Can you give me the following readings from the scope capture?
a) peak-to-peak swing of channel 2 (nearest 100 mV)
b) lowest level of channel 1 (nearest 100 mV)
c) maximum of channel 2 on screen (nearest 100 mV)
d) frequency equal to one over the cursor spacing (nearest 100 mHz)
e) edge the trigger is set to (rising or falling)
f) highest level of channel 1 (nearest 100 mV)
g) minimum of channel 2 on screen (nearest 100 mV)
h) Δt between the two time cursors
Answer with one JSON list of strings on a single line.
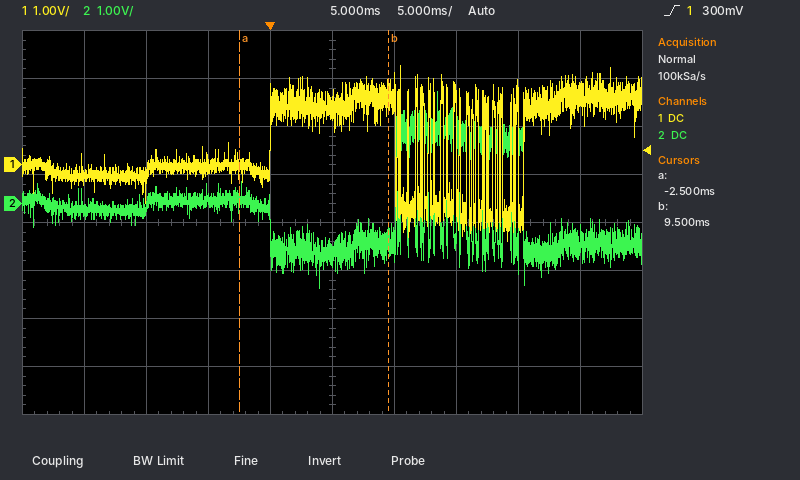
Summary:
["4.1 V", "-1.6 V", "2.3 V", "83.3 Hz", "rising", "2.1 V", "-1.8 V", "12.0 ms"]
